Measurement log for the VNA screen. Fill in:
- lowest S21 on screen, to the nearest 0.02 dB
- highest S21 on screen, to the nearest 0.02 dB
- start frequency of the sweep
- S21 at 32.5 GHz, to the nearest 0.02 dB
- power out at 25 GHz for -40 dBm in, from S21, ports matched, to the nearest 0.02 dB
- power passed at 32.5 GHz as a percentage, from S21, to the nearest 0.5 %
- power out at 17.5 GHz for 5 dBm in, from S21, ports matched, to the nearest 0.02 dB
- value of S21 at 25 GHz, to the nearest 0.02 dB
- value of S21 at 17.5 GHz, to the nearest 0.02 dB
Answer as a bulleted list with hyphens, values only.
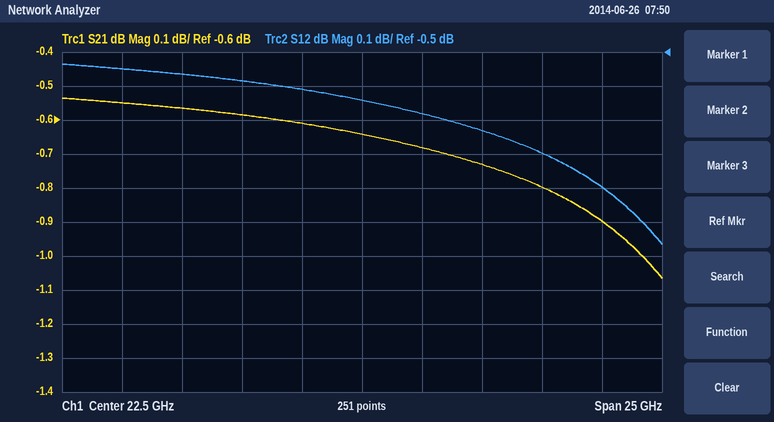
- -1.06 dB
- -0.54 dB
- 10 GHz
- -0.90 dB
- -40.68 dBm
- 81.5 %
- 4.42 dBm
- -0.68 dB
- -0.58 dB
